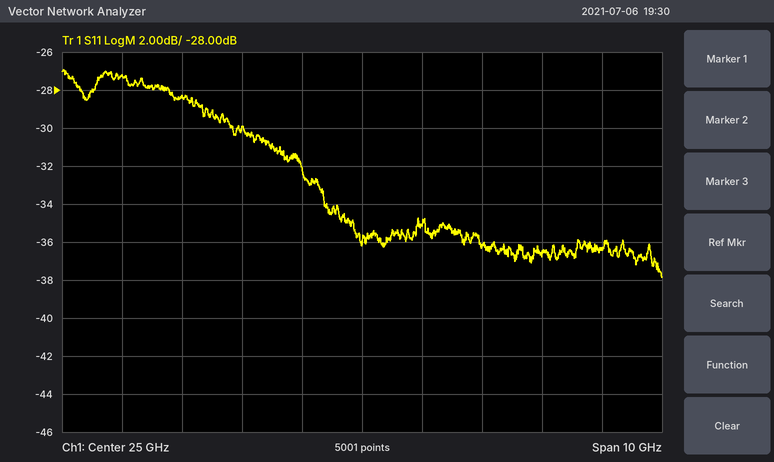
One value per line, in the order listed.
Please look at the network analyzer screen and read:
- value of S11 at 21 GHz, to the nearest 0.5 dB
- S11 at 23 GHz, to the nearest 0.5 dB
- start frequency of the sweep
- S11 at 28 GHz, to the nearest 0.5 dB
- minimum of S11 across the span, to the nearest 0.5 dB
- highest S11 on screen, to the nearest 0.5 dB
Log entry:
-27.0 dB
-30.0 dB
20 GHz
-36.5 dB
-38.0 dB
-27.0 dB
